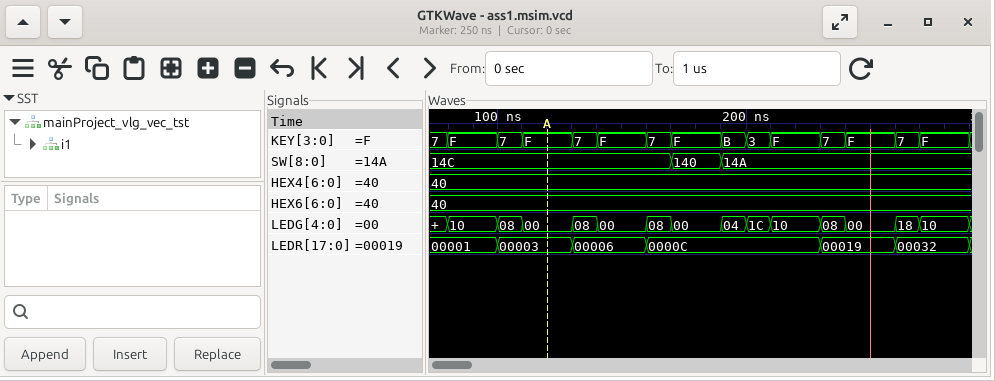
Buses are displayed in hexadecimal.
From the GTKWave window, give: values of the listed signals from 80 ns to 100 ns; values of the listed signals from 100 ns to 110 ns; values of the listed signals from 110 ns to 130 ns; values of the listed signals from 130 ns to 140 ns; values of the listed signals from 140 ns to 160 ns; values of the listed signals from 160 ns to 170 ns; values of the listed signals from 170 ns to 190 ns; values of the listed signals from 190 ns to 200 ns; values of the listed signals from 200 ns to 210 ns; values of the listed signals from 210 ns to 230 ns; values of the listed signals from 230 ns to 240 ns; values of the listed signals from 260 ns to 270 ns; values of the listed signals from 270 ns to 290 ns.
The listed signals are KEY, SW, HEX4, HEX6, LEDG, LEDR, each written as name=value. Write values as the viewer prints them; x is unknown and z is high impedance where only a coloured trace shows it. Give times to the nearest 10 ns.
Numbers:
KEY=F, SW=14C, HEX4=40, HEX6=40, LEDG=10, LEDR=00001
KEY=7, SW=14C, HEX4=40, HEX6=40, LEDG=08, LEDR=00003
KEY=F, SW=14C, HEX4=40, HEX6=40, LEDG=00, LEDR=00003
KEY=7, SW=14C, HEX4=40, HEX6=40, LEDG=08, LEDR=00006
KEY=F, SW=14C, HEX4=40, HEX6=40, LEDG=00, LEDR=00006
KEY=7, SW=14C, HEX4=40, HEX6=40, LEDG=08, LEDR=0000C
KEY=F, SW=140, HEX4=40, HEX6=40, LEDG=00, LEDR=0000C
KEY=B, SW=14A, HEX4=40, HEX6=40, LEDG=04, LEDR=0000C
KEY=3, SW=14A, HEX4=40, HEX6=40, LEDG=1C, LEDR=0000C
KEY=F, SW=14A, HEX4=40, HEX6=40, LEDG=10, LEDR=0000C
KEY=7, SW=14A, HEX4=40, HEX6=40, LEDG=08, LEDR=00019
KEY=7, SW=14A, HEX4=40, HEX6=40, LEDG=18, LEDR=00032
KEY=F, SW=14A, HEX4=40, HEX6=40, LEDG=10, LEDR=00032
